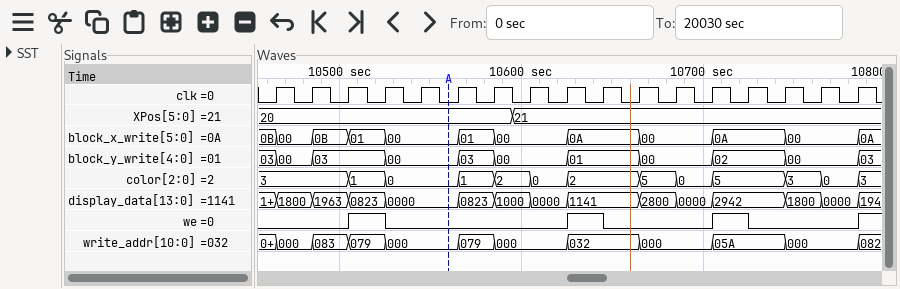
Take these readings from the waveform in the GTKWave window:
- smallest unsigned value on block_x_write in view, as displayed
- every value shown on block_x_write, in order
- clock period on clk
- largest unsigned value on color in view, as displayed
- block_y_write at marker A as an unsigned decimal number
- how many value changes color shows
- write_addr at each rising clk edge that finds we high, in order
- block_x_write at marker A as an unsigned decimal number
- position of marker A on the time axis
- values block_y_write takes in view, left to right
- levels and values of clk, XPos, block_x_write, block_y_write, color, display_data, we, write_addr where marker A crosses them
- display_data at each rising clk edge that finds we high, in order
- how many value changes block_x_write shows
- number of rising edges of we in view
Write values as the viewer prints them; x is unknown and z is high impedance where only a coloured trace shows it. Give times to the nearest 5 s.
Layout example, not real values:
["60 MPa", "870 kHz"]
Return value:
["00", "0B, 00, 0B, 01, 00, 01, 00, 0A, 00, 0A, 00, 0A", "20 s", "5", "0", "12", "079, 032, 05A", "0", "10560 s", "03, 00, 03, 00, 03, 00, 01, 00, 02, 00, 03", "clk=0, XPos=20, block_x_write=00, block_y_write=00, color=0, display_data=0000, we=0, write_addr=000", "0823, 1141, 2942", "11", "4"]
